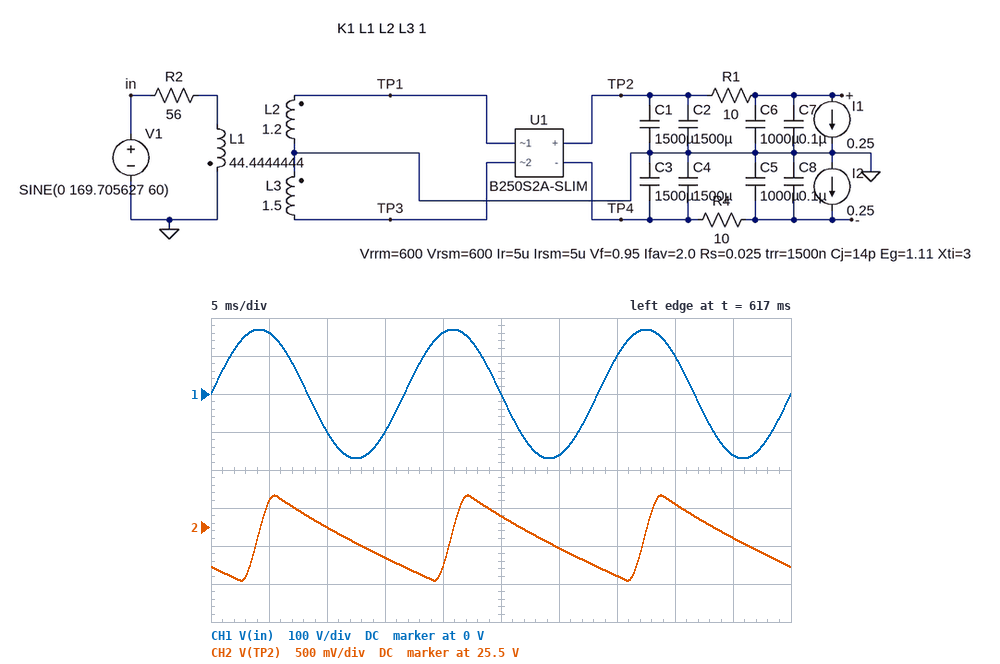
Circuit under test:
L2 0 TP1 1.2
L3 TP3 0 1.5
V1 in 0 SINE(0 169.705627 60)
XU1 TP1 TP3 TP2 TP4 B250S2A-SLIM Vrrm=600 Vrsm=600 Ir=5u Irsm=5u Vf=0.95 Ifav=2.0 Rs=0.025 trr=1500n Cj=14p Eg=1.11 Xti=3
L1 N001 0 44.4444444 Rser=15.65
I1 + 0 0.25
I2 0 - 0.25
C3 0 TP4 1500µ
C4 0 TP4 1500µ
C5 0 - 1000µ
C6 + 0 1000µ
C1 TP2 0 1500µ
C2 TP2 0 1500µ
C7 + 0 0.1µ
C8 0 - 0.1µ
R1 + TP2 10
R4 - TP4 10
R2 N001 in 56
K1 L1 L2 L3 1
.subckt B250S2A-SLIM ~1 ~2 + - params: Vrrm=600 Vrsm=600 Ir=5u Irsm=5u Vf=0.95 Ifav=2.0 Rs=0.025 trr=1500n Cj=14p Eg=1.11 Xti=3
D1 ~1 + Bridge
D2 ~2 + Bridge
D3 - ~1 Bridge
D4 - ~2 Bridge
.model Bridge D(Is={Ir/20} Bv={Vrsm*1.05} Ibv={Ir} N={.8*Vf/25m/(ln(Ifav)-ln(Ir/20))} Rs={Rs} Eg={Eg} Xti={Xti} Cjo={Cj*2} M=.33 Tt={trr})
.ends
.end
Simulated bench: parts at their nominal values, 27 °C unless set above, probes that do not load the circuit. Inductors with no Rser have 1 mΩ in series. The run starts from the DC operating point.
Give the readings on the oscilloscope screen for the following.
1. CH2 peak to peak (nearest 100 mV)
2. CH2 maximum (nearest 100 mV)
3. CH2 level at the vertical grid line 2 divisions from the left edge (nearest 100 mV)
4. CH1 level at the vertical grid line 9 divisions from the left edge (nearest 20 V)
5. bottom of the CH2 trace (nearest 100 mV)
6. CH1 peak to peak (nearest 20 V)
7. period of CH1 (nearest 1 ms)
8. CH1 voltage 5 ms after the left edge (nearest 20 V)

1.1 V
25.9 V
25.5 V
-160 V
24.8 V
340 V
17 ms
160 V
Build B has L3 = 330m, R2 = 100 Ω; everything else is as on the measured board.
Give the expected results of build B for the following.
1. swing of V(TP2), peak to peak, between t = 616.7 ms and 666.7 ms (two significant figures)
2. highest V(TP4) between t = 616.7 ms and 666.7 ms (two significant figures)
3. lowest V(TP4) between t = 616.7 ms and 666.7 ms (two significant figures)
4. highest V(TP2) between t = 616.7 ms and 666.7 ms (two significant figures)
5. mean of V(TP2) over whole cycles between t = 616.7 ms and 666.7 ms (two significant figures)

1.1 V
-21 V
-22 V
22 V
21 V
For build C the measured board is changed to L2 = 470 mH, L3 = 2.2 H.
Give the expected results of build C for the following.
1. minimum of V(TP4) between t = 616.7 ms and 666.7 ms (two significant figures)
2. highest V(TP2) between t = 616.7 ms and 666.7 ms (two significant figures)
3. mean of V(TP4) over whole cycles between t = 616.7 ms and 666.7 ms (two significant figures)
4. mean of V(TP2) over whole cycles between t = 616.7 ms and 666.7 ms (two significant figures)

-31 V
31 V
-30 V
30 V
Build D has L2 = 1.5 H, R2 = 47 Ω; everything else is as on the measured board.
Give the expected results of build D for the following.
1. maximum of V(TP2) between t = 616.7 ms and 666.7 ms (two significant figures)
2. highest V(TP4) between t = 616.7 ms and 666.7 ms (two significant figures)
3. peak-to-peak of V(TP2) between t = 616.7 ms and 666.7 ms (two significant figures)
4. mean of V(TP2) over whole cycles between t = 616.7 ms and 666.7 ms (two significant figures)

26 V
-26 V
460 mV
26 V
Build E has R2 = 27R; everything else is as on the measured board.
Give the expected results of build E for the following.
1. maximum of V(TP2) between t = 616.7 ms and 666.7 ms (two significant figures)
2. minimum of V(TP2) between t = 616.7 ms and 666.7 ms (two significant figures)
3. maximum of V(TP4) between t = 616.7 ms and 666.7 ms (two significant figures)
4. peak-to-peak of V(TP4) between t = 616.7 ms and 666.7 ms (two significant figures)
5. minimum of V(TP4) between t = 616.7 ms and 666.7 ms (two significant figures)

27 V
26 V
-26 V
1.2 V
-27 V
